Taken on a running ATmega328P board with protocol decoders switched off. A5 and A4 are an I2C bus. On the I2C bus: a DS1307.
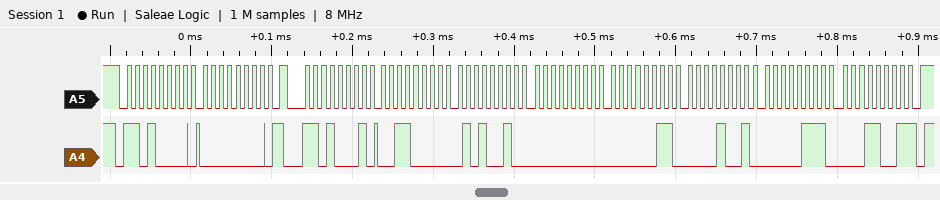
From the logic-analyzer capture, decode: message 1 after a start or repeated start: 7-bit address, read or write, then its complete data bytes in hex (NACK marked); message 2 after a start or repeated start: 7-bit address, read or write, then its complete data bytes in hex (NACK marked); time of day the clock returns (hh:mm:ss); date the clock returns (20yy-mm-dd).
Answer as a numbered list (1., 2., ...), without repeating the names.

1. 0x68 write: 00
2. 0x68 read: 30 52 00 03 09 07 19 NACK
3. 00:52:30
4. 2019-07-09
